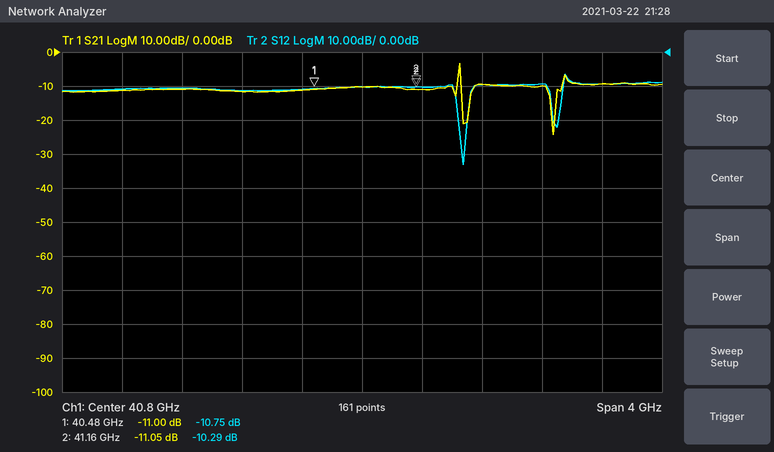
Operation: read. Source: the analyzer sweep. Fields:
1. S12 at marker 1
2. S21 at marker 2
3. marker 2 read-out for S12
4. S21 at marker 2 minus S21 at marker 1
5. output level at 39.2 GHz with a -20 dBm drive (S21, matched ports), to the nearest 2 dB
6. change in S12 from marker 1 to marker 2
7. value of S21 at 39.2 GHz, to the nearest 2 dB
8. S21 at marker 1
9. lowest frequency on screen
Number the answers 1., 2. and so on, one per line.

1. -10.75 dB
2. -11.05 dB
3. -10.29 dB
4. -0.05 dB
5. -32 dBm
6. 0.46 dB
7. -12 dB
8. -11.00 dB
9. 38.8 GHz
